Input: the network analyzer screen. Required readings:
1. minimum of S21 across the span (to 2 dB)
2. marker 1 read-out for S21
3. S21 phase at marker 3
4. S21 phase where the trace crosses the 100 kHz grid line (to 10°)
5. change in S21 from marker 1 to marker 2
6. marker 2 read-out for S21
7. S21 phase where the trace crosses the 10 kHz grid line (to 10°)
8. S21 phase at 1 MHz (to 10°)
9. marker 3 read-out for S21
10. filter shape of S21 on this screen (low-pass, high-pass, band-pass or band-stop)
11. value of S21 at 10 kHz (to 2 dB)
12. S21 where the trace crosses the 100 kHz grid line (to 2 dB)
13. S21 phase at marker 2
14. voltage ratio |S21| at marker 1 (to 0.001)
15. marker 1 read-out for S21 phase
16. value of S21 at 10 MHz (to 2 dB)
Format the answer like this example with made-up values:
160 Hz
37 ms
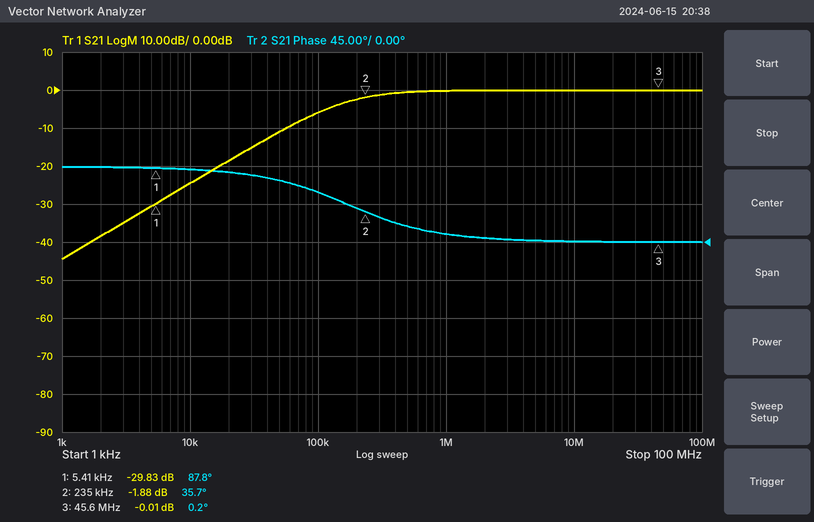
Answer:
-44 dB
-29.83 dB
0.2°
60°
27.95 dB
-1.88 dB
90°
10°
-0.01 dB
high-pass
-24 dB
-6 dB
35.7°
0.032
87.8°
0 dB
